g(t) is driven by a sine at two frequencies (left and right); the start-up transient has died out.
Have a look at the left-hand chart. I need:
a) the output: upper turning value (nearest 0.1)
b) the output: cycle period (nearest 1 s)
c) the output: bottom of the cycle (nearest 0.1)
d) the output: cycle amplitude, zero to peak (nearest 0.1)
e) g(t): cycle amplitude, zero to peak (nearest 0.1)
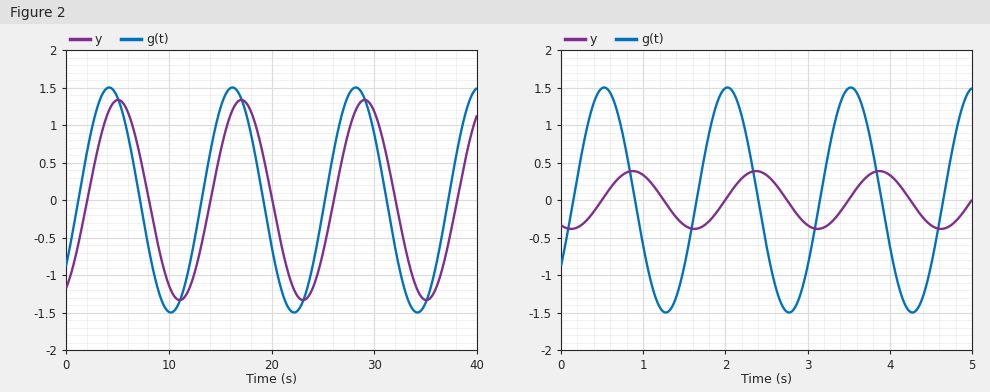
1.3
12 s
-1.3
1.3
1.5
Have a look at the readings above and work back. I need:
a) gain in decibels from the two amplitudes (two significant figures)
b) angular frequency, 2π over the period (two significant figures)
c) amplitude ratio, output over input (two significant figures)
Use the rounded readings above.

-1.2 dB
0.52 rad/s
0.87
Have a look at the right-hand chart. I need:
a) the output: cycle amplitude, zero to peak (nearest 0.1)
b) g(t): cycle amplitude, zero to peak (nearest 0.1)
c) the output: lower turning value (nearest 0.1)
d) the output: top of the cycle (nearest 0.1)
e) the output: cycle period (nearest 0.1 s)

0.4
1.5
-0.4
0.4
1.5 s
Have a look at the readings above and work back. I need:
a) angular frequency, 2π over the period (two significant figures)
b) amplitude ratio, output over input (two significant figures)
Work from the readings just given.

4.2 rad/s
0.27
